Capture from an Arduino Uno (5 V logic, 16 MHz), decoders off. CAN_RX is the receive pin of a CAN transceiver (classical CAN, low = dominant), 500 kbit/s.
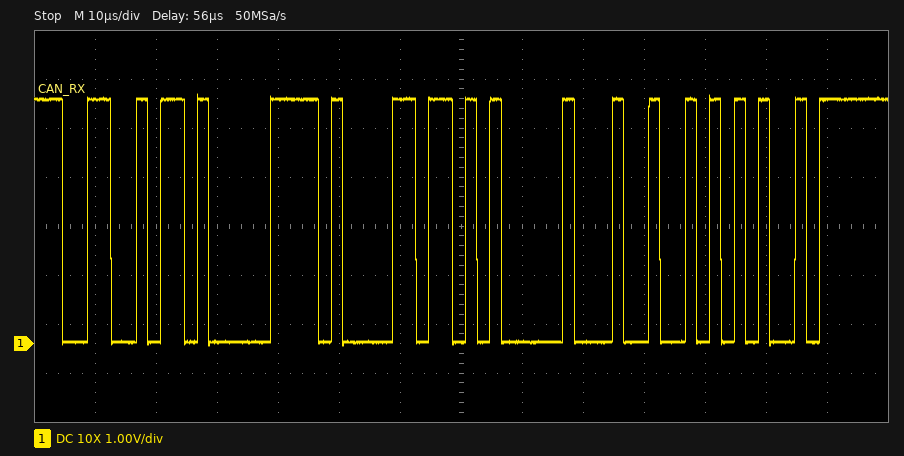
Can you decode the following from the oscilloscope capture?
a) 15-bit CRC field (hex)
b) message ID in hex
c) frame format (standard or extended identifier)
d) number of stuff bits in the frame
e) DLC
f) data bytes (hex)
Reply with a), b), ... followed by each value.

a) 0x4954
b) 0x32D
c) standard
d) 2
e) 3
f) A1 B5 00
